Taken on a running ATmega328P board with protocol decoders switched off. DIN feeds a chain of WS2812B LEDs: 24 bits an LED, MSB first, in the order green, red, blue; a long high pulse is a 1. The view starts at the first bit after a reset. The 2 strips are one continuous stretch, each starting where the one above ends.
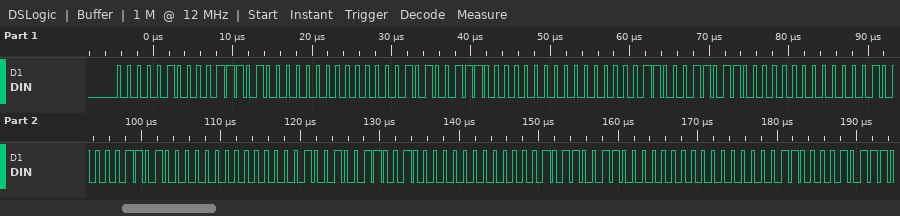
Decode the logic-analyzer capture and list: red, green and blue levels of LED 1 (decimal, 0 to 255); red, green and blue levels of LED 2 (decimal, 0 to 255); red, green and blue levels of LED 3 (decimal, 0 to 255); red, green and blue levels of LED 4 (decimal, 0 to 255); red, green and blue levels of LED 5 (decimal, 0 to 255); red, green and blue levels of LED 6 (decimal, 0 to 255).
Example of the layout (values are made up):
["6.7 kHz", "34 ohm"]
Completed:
["58, 4, 0", "56, 5, 0", "54, 6, 0", "52, 8, 0", "50, 9, 0", "48, 11, 0"]
